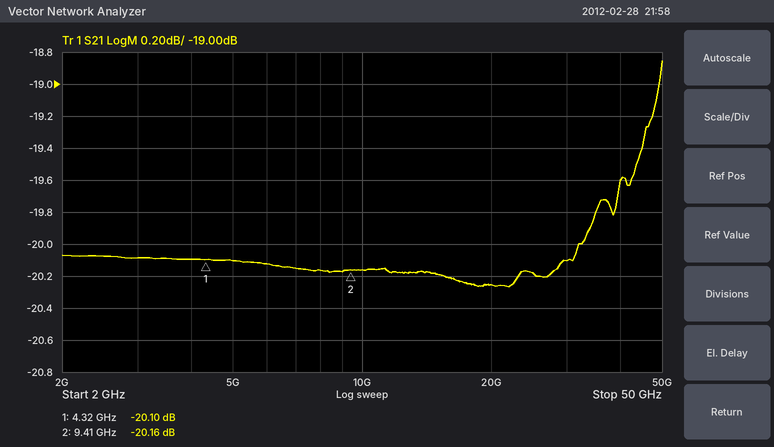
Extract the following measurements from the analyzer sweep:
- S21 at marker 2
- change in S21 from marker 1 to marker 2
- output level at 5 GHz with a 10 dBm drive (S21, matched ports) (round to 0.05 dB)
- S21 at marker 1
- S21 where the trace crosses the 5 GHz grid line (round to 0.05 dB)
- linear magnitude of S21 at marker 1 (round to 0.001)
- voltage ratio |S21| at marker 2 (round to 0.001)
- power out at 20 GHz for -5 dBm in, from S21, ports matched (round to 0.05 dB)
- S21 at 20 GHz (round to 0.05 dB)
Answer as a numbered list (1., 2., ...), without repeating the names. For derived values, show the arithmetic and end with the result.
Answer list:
1. -20.16 dB
2. -20.16 − (-20.1) = -0.06 dB
3. 10 dBm + (-20.10 dB) = -10.10 dBm
4. -20.10 dB
5. -20.10 dB
6. 10^(-20.1/20) ≈ 0.099
7. 10^(-20.16/20) ≈ 0.098
8. -5 dBm + (-20.25 dB) = -25.25 dBm
9. -20.25 dB
